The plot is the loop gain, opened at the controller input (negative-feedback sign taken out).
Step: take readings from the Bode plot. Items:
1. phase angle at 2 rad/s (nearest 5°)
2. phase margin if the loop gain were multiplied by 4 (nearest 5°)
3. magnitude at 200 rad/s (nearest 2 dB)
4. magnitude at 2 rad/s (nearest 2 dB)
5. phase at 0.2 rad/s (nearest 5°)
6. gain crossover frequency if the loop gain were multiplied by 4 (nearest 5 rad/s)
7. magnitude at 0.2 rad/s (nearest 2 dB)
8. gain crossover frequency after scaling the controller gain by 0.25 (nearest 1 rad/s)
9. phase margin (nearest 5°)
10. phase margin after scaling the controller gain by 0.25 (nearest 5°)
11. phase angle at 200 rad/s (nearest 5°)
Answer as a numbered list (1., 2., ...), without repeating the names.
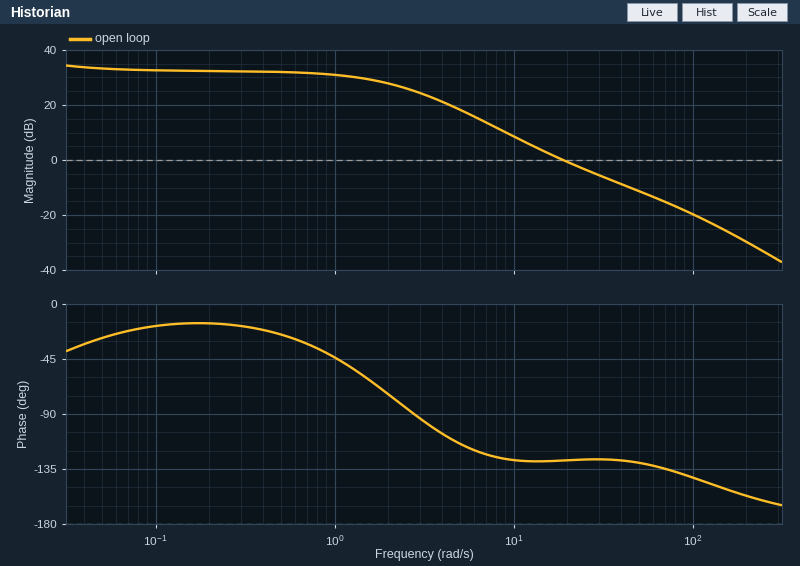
1. -75°
2. 50°
3. -30 dB
4. 28 dB
5. -15°
6. 55 rad/s
7. 32 dB
8. 8 rad/s
9. 50°
10. 55°
11. -155°
